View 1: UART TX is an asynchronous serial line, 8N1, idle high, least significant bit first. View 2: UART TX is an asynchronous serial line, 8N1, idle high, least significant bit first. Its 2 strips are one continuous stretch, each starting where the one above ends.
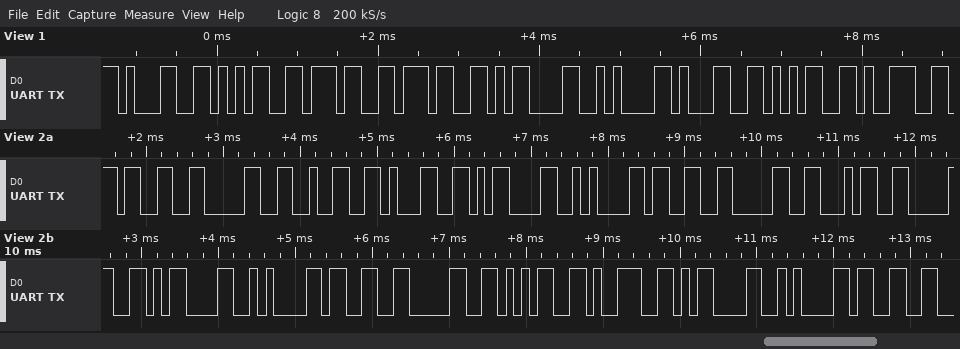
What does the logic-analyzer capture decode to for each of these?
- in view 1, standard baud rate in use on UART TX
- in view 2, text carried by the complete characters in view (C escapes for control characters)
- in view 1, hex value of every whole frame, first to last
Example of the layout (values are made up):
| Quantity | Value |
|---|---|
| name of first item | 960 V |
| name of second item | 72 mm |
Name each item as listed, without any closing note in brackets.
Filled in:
| Quantity | Value |
|---|---|
| in view 1, standard baud rate in use on UART TX | 9600 baud |
| in view 2, text carried by the complete characters in view | "3021\r\n3040\r\n3059\r\n3" |
| in view 1, hex value of every whole frame, first to last | 0x31 0x35 0x37 0x37 0x0D 0x0A 0x31 0x35 0x39 |
